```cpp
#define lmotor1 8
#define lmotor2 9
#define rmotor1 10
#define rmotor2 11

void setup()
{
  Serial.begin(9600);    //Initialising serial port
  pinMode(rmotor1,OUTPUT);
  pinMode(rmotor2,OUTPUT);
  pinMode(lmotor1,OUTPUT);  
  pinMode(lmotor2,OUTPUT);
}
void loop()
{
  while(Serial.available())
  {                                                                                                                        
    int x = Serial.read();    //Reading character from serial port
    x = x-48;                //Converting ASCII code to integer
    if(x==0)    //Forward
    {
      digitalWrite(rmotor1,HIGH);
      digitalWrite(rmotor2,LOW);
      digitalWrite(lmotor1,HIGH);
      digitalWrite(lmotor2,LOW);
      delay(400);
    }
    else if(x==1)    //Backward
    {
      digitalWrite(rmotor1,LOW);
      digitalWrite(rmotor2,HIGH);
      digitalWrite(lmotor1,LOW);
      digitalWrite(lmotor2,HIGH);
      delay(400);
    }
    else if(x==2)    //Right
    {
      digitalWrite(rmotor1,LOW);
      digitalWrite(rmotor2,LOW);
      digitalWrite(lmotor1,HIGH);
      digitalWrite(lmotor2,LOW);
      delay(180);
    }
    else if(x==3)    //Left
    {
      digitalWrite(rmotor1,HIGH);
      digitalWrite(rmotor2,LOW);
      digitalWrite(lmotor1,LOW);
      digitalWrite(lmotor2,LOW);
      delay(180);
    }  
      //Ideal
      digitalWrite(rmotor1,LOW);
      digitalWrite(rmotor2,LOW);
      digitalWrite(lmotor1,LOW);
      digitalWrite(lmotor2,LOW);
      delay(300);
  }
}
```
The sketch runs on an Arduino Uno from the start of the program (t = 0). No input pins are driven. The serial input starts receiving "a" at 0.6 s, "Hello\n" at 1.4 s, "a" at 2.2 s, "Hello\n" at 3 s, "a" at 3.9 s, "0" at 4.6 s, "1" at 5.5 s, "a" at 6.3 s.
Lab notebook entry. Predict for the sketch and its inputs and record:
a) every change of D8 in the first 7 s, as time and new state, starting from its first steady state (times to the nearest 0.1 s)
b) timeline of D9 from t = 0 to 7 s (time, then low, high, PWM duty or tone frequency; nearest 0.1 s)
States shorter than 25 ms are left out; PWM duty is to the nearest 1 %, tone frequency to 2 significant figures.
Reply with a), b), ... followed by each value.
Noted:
a) 0 s low; 5.6 s high; 6 s low
b) 0 s low; 6.3 s high; 6.7 s low
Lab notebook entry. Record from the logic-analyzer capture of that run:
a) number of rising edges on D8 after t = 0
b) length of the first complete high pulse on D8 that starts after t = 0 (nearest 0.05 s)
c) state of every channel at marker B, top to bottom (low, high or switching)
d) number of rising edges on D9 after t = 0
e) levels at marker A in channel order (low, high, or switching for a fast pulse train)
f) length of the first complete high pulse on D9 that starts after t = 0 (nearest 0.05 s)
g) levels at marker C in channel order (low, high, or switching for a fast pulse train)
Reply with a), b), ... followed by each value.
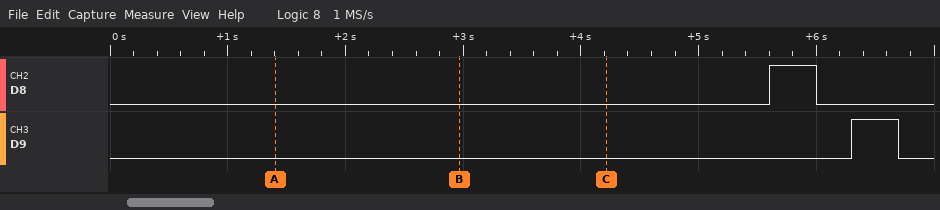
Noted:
a) 1
b) 0.40 s
c) D8 low, D9 low
d) 1
e) D8 low, D9 low
f) 0.40 s
g) D8 low, D9 low
